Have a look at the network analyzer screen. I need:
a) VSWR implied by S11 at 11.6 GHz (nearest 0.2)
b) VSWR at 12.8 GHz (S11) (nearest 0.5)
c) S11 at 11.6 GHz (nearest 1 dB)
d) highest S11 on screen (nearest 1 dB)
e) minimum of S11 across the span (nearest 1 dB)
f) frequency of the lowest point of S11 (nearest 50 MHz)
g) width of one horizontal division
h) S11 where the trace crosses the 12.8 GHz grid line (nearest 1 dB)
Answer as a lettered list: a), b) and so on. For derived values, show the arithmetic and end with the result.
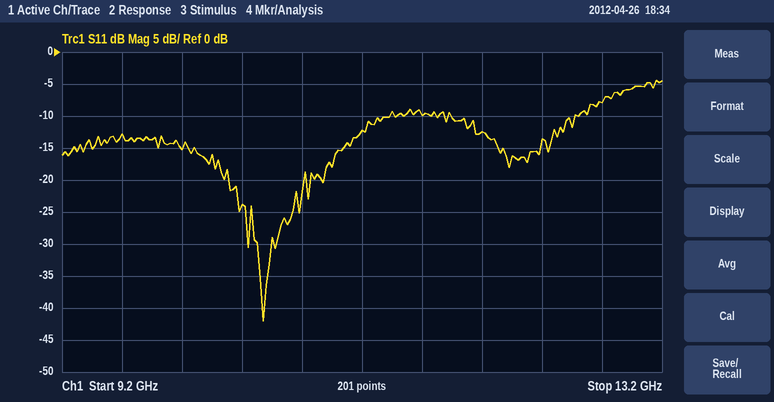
a) |Γ| = 10^(-10/20) = 0.3162; VSWR = (1 + 0.3162)/(1 − 0.3162) ≈ 1.92, so 2.0 to the nearest 0.2
b) |Γ| = 10^(-8/20) = 0.3981; VSWR = (1 + 0.3981)/(1 − 0.3981) ≈ 2.32, so 2.5 to the nearest 0.5
c) -10 dB
d) -4 dB
e) -42 dB
f) 10.55 GHz
g) 400 MHz
h) -8 dB
